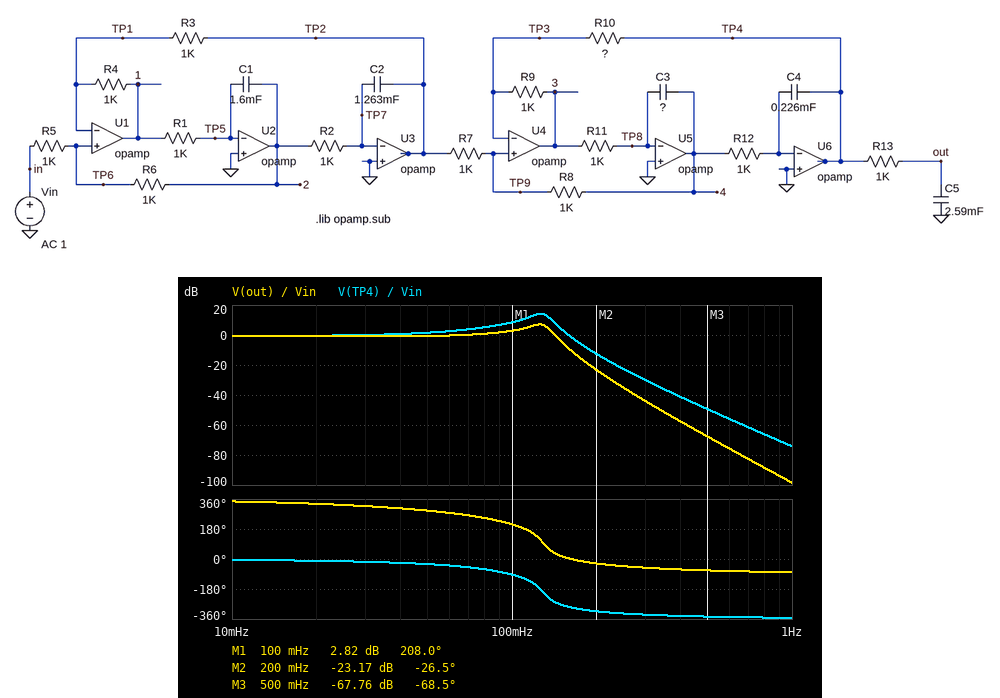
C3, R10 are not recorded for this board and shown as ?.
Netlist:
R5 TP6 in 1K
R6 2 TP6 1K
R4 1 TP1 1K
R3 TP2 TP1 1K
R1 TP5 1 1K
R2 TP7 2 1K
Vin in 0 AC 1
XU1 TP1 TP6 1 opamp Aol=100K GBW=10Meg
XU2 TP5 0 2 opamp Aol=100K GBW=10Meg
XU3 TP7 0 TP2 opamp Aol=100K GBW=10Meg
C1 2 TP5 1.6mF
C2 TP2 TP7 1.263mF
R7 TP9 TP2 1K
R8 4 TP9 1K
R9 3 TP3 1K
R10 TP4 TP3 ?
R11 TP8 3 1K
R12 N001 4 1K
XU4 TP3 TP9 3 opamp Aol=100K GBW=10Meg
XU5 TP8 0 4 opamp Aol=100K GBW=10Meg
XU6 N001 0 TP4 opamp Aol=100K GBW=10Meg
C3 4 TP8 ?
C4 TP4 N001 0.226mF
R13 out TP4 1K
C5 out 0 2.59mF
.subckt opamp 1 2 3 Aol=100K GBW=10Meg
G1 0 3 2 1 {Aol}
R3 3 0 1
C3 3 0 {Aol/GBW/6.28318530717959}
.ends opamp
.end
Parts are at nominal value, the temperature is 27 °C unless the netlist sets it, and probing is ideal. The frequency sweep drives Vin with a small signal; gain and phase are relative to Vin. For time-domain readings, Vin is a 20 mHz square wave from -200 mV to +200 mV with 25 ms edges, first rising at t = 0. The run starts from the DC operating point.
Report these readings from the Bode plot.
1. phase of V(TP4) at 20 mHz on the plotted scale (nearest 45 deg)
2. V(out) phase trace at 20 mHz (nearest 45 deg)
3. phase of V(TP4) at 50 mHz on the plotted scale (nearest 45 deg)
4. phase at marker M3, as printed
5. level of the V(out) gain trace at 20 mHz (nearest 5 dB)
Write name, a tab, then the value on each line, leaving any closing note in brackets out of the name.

phase of V(TP4) at 20 mHz on the plotted scale	0 deg
V(out) phase trace at 20 mHz	315 deg
phase of V(TP4) at 50 mHz on the plotted scale	-45 deg
phase at marker M3, as printed	-68.5 deg
level of the V(out) gain trace at 20 mHz	0 dB
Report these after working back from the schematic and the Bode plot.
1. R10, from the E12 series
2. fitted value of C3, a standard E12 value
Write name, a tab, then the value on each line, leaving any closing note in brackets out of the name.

R10, from the E12 series	820 Ω
fitted value of C3, a standard E12 value	8.2 mF
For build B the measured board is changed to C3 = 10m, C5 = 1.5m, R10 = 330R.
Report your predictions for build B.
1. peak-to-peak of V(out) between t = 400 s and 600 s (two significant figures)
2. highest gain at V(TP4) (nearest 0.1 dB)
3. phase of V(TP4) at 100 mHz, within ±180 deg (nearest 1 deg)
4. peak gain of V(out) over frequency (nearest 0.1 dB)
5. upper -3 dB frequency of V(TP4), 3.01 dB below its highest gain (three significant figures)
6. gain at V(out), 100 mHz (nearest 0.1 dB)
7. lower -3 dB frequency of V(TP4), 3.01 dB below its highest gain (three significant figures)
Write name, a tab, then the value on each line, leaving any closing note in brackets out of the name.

peak-to-peak of V(out) between t = 400 s and 600 s	430 mV
highest gain at V(TP4)	5.0 dB
phase of V(TP4) at 100 mHz, within ±180 deg	-83 deg
peak gain of V(out) over frequency	-0.9 dB
upper -3 dB frequency of V(TP4), 3.01 dB below its highest gain	194 mHz
gain at V(out), 100 mHz	-1.6 dB
lower -3 dB frequency of V(TP4), 3.01 dB below its highest gain	148 mHz
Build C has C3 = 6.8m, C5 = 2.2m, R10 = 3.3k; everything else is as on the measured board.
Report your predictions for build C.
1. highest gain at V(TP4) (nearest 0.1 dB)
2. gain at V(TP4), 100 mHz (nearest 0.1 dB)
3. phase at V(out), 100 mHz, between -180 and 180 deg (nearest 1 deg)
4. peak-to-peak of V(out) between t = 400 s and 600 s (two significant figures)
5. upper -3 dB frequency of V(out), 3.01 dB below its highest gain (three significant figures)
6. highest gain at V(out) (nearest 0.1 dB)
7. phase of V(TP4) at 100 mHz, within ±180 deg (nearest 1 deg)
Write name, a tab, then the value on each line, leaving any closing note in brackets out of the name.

highest gain at V(TP4)	21.7 dB
gain at V(TP4), 100 mHz	8.0 dB
phase at V(out), 100 mHz, between -180 and 180 deg	67 deg
peak-to-peak of V(out) between t = 400 s and 600 s	1.9 V
upper -3 dB frequency of V(out), 3.01 dB below its highest gain	76.8 mHz
highest gain at V(out)	18.8 dB
phase of V(TP4) at 100 mHz, within ±180 deg	121 deg
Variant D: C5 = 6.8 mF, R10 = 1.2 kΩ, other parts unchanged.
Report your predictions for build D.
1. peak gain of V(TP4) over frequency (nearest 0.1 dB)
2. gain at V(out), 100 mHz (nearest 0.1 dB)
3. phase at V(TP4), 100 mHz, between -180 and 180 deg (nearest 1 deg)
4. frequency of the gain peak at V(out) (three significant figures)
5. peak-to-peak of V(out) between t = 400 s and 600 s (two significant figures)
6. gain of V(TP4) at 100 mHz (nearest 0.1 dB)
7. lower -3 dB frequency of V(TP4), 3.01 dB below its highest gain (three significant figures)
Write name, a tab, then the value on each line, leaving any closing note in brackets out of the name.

peak gain of V(TP4) over frequency	17.9 dB
gain at V(out), 100 mHz	3.8 dB
phase at V(TP4), 100 mHz, between -180 and 180 deg	-128 deg
frequency of the gain peak at V(out)	105 mHz
peak-to-peak of V(out) between t = 400 s and 600 s	490 mV
gain of V(TP4) at 100 mHz	16.6 dB
lower -3 dB frequency of V(TP4), 3.01 dB below its highest gain	95.7 mHz
